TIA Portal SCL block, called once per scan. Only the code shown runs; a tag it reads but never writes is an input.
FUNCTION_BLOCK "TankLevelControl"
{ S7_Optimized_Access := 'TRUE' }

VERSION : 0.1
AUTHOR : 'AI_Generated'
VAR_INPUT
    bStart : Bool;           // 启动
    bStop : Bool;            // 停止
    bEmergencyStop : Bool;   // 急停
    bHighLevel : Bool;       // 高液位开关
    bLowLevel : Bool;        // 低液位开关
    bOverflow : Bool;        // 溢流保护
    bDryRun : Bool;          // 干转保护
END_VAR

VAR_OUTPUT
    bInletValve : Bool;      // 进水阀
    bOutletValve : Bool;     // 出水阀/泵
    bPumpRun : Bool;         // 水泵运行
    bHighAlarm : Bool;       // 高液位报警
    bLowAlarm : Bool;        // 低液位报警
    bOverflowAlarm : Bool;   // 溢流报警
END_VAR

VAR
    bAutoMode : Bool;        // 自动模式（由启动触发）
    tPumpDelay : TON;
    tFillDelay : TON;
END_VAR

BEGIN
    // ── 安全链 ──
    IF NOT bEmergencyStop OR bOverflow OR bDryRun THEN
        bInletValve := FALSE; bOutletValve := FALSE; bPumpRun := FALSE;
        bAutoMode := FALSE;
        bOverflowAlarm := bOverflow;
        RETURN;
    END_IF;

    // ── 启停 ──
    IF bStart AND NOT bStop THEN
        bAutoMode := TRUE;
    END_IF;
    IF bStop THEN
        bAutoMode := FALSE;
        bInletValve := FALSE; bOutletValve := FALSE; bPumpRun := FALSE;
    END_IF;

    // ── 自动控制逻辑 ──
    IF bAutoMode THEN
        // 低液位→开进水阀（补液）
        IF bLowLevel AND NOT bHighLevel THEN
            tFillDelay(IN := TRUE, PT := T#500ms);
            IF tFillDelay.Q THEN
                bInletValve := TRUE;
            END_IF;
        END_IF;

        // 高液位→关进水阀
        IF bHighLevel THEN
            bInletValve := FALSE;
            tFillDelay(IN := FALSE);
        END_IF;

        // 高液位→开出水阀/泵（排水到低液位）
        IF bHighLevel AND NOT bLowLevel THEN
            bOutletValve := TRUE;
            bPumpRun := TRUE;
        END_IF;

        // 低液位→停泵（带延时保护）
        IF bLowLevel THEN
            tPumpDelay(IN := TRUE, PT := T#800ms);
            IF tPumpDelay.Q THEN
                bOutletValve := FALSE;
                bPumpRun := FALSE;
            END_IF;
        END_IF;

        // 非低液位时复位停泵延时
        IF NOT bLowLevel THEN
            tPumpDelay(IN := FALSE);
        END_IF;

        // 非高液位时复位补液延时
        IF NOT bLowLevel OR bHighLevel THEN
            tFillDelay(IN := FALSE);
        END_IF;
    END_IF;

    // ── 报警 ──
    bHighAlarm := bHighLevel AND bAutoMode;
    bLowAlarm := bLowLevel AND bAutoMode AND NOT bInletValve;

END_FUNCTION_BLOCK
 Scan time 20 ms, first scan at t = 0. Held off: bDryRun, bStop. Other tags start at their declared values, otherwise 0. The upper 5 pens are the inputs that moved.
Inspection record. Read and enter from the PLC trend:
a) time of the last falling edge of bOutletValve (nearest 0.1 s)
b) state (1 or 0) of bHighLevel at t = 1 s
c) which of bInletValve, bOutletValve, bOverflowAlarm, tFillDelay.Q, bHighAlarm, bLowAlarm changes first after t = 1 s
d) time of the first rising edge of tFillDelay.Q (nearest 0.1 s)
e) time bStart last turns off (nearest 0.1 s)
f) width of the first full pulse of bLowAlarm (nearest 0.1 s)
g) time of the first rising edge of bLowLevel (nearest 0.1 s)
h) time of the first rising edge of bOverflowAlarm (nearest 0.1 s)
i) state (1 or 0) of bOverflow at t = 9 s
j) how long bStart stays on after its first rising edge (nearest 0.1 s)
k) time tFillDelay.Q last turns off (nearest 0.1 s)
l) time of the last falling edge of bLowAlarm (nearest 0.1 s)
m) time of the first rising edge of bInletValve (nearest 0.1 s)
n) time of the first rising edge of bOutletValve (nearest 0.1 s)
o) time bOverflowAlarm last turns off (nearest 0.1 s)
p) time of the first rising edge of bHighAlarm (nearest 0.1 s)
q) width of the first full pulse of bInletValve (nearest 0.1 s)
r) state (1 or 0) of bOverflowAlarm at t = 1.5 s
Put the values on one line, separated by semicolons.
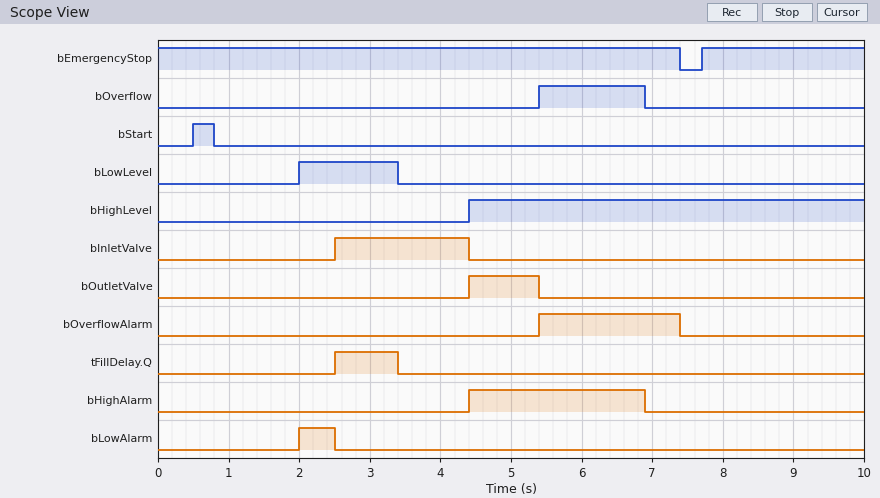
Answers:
5.4 s; 0; bLowAlarm; 2.5 s; 0.8 s; 0.5 s; 2.0 s; 5.4 s; 0; 0.3 s; 3.4 s; 2.5 s; 2.5 s; 4.4 s; 7.4 s; 4.4 s; 1.9 s; 0
